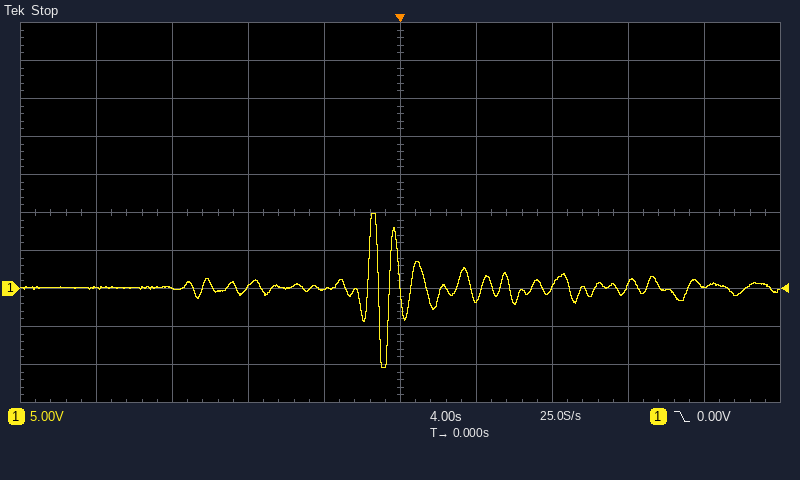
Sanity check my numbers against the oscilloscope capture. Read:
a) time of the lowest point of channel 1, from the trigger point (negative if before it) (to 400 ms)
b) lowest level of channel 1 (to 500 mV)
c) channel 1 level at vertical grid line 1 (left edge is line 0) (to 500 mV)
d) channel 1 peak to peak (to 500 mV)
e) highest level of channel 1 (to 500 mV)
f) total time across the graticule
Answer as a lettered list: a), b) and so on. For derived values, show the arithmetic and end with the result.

a) -800 ms
b) -10.5 V
c) 0.0 V
d) 10.0 V − (-10.5 V) = 20.5 V
e) 10.0 V
f) 40 s
